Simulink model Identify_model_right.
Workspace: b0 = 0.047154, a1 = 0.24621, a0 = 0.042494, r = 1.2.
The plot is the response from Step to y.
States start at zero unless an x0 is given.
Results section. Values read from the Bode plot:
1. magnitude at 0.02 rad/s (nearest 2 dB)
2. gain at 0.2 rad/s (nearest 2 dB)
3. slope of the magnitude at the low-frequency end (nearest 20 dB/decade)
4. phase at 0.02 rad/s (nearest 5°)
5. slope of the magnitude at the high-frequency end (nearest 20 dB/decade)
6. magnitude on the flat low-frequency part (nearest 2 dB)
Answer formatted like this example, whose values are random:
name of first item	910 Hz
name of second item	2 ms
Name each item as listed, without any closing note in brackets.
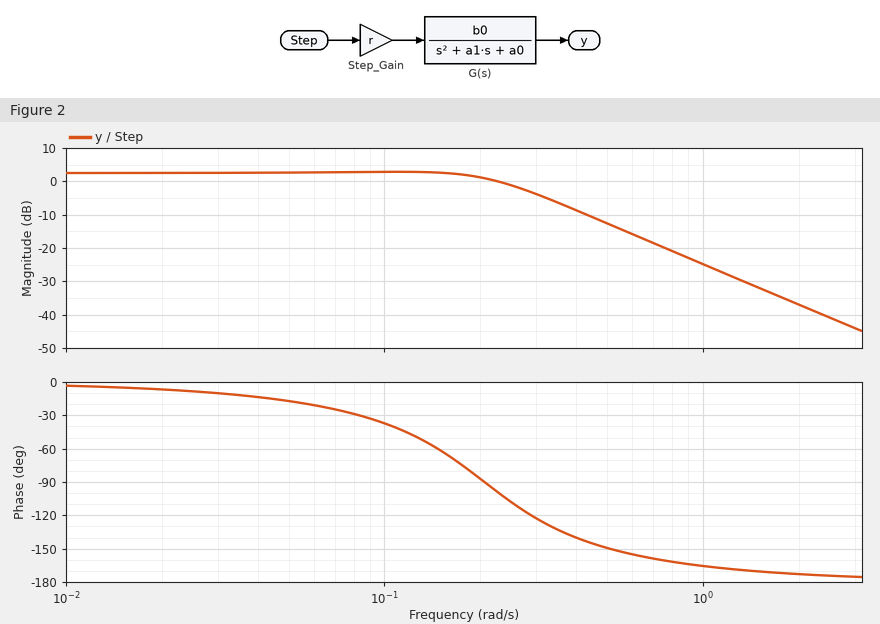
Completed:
magnitude at 0.02 rad/s	2 dB
gain at 0.2 rad/s	2 dB
slope of the magnitude at the low-frequency end	0 dB/decade
phase at 0.02 rad/s	-5°
slope of the magnitude at the high-frequency end	-40 dB/decade
magnitude on the flat low-frequency part	2 dB
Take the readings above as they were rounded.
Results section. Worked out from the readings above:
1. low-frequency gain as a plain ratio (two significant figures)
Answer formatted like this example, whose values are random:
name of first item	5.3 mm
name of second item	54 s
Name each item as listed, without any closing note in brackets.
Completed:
low-frequency gain as a plain ratio	1.3
